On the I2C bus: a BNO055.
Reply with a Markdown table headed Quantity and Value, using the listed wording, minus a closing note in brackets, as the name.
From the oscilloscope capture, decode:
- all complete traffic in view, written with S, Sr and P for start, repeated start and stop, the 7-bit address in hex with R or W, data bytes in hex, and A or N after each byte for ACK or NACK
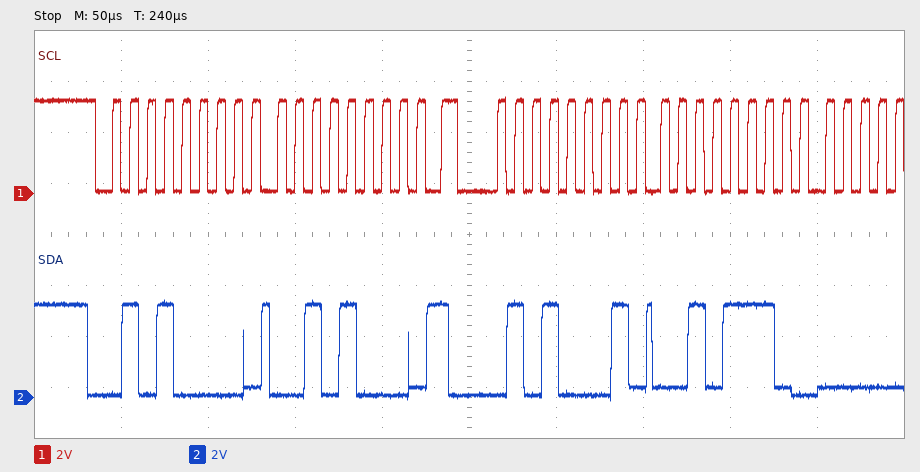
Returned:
| Quantity | Value |
|---|---|
| all complete traffic in view, written with S, Sr and P for start, repeated start and stop, the 7-bit address in hex with R or W, data bytes in hex, and A or N after each byte for ACK or NACK | S 28W A 28 A Sr 28R A 2E A |
